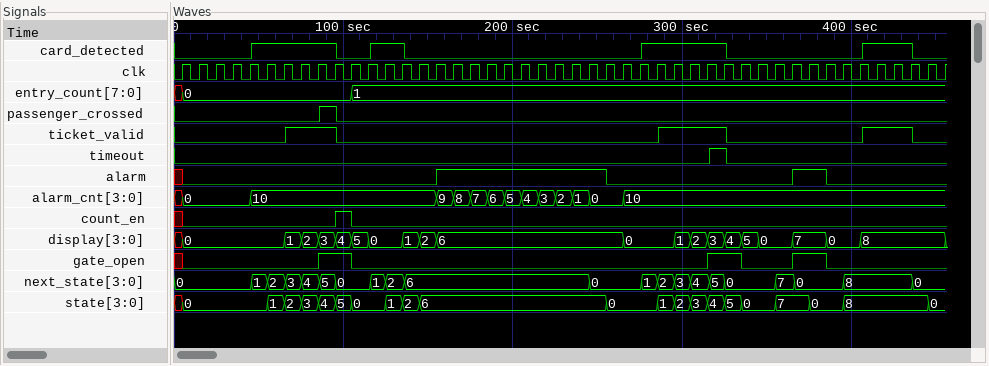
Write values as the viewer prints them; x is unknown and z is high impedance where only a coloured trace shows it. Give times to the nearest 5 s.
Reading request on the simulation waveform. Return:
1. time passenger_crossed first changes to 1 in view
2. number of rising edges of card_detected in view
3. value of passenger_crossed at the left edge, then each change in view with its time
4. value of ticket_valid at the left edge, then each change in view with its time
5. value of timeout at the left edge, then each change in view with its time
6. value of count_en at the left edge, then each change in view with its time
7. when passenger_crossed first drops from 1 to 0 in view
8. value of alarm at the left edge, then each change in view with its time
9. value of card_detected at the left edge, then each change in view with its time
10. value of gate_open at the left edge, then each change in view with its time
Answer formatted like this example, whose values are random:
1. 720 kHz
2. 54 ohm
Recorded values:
1. 85 s
2. 4
3. 0, 1 at 85 s, 0 at 95 s
4. 0, 1 at 65 s, 0 at 95 s, 1 at 285 s, 0 at 325 s, 1 at 405 s, 0 at 435 s
5. 0, 1 at 315 s, 0 at 325 s
6. x, 0 at 5 s, 1 at 95 s, 0 at 105 s
7. 95 s
8. x, 0 at 5 s, 1 at 155 s, 0 at 255 s, 1 at 365 s, 0 at 385 s
9. 0, 1 at 45 s, 0 at 95 s, 1 at 115 s, 0 at 135 s, 1 at 275 s, 0 at 325 s, 1 at 405 s, 0 at 435 s
10. x, 0 at 5 s, 1 at 85 s, 0 at 105 s, 1 at 315 s, 0 at 335 s, 1 at 365 s, 0 at 385 s
